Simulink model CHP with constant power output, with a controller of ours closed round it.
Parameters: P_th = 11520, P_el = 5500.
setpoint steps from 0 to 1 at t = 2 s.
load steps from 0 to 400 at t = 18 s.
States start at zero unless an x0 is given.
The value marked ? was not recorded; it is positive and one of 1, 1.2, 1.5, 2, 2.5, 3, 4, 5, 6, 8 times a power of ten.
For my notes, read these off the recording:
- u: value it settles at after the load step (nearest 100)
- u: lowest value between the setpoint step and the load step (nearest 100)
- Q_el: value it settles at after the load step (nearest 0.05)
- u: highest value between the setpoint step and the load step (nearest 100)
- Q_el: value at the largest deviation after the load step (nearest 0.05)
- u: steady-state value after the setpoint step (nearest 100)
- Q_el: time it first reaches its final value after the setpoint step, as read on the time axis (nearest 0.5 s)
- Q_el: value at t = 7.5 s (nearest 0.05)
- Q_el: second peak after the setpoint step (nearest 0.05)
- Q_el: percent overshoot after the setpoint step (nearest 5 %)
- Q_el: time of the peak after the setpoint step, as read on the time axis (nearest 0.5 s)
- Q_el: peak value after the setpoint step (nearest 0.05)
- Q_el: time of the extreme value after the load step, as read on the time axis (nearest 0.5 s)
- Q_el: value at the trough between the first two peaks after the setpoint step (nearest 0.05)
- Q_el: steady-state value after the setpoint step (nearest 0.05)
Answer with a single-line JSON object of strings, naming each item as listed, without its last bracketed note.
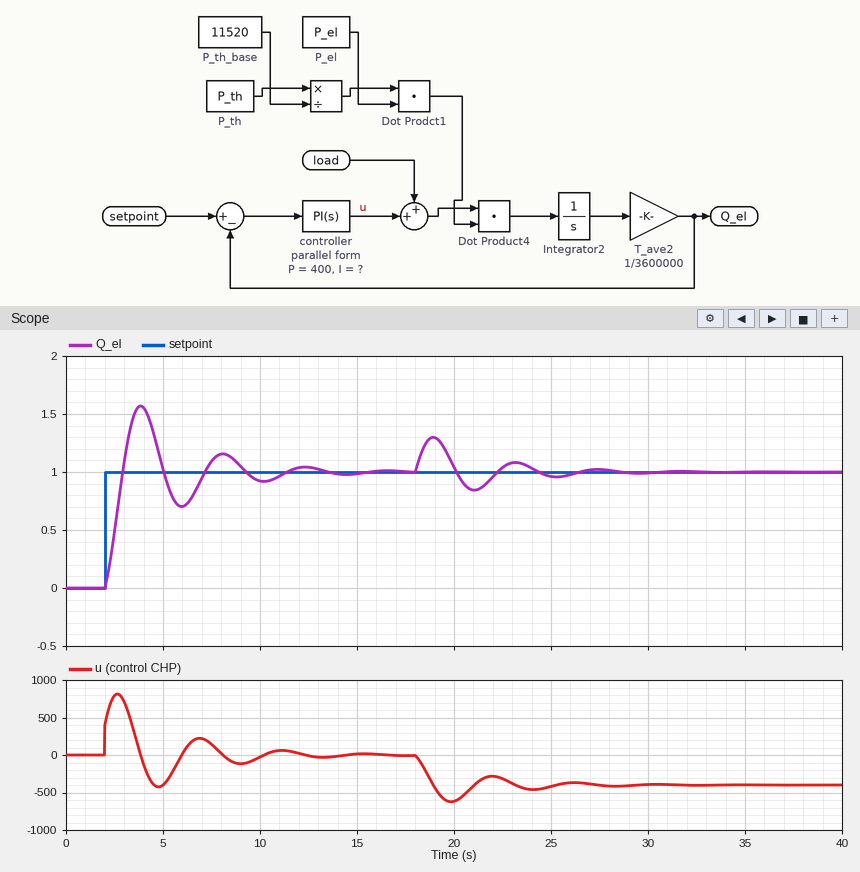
{"u: value it settles at after the load step": "-400", "u: lowest value between the setpoint step and the load step": "-400", "Q_el: value it settles at after the load step": "1.00", "u: highest value between the setpoint step and the load step": "800", "Q_el: value at the largest deviation after the load step": "1.30", "u: steady-state value after the setpoint step": "0", "Q_el: time it first reaches its final value after the setpoint step, as read on the time axis": "3.0 s", "Q_el: value at t = 7.5 s": "1.10", "Q_el: second peak after the setpoint step": "1.15", "Q_el: percent overshoot after the setpoint step": "55 %", "Q_el: time of the peak after the setpoint step, as read on the time axis": "4.0 s", "Q_el: peak value after the setpoint step": "1.55", "Q_el: time of the extreme value after the load step, as read on the time axis": "19.0 s", "Q_el: value at the trough between the first two peaks after the setpoint step": "0.70", "Q_el: steady-state value after the setpoint step": "1.00"}
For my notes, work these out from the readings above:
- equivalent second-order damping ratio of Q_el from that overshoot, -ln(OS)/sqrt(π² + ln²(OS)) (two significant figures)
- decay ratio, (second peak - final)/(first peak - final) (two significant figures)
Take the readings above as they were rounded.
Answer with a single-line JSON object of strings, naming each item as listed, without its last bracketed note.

{"equivalent second-order damping ratio of Q_el from that overshoot, -ln(OS)/sqrt(π² + ln²(OS))": "0.19", "decay ratio, (second peak - final)/(first peak - final)": "0.27"}
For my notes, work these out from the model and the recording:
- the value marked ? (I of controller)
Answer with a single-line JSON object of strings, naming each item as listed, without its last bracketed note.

{"the value marked ?": "1500"}
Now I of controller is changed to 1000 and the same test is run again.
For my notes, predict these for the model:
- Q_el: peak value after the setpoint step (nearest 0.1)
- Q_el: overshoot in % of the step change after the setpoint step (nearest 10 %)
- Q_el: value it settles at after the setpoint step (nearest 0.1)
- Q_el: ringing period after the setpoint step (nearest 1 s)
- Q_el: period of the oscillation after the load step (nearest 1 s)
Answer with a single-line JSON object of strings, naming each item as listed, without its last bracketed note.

{"Q_el: peak value after the setpoint step": "1.5", "Q_el: overshoot in % of the step change after the setpoint step": "50 %", "Q_el: value it settles at after the setpoint step": "1.0", "Q_el: ringing period after the setpoint step": "5 s", "Q_el: period of the oscillation after the load step": "5 s"}
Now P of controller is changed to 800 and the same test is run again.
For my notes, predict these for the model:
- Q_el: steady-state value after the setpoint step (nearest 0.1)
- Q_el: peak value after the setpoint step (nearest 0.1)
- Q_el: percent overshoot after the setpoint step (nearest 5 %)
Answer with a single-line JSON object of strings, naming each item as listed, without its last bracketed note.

{"Q_el: steady-state value after the setpoint step": "1.0", "Q_el: peak value after the setpoint step": "1.4", "Q_el: percent overshoot after the setpoint step": "35 %"}
